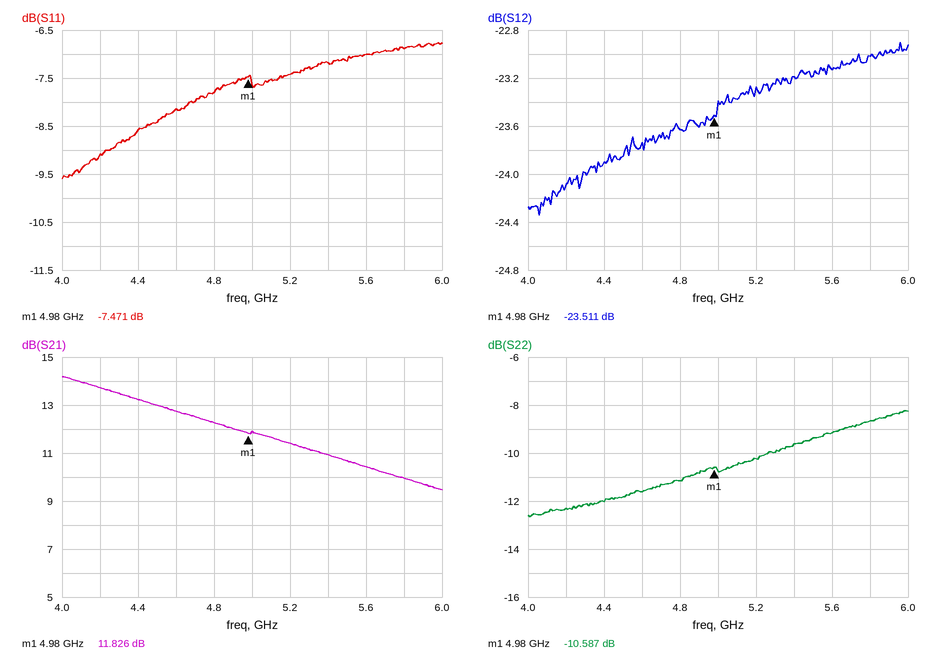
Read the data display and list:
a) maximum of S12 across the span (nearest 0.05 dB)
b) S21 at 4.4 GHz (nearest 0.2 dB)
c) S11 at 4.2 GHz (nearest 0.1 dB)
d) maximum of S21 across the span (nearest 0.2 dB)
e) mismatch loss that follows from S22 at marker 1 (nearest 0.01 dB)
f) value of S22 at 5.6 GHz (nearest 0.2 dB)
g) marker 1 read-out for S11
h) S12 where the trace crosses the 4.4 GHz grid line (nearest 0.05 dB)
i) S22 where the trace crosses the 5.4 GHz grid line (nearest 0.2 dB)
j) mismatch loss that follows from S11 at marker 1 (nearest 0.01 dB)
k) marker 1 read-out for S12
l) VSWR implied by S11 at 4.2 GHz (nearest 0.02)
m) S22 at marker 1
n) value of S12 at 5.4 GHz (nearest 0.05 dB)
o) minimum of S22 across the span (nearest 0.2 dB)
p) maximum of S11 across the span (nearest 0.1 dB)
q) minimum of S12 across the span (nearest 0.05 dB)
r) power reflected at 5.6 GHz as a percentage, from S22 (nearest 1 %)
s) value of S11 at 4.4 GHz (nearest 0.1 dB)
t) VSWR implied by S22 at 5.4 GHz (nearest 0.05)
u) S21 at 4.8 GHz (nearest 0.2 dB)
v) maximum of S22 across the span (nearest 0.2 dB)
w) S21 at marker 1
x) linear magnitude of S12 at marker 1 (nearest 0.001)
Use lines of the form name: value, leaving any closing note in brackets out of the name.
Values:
maximum of S12 across the span: -22.90 dB
S21 at 4.4 GHz: 13.2 dB
S11 at 4.2 GHz: -9.1 dB
maximum of S21 across the span: 14.2 dB
mismatch loss that follows from S22 at marker 1: 0.40 dB
value of S22 at 5.6 GHz: -9.2 dB
marker 1 read-out for S11: -7.471 dB
S12 where the trace crosses the 4.4 GHz grid line: -23.90 dB
S22 where the trace crosses the 5.4 GHz grid line: -9.6 dB
mismatch loss that follows from S11 at marker 1: 0.86 dB
marker 1 read-out for S12: -23.511 dB
VSWR implied by S11 at 4.2 GHz: 2.08
S22 at marker 1: -10.587 dB
value of S12 at 5.4 GHz: -23.20 dB
minimum of S22 across the span: -12.6 dB
maximum of S11 across the span: -6.8 dB
minimum of S12 across the span: -24.35 dB
power reflected at 5.6 GHz as a percentage, from S22: 12 %
value of S11 at 4.4 GHz: -8.6 dB
VSWR implied by S22 at 5.4 GHz: 2.00
S21 at 4.8 GHz: 12.2 dB
maximum of S22 across the span: -8.2 dB
S21 at marker 1: 11.826 dB
linear magnitude of S12 at marker 1: 0.067
